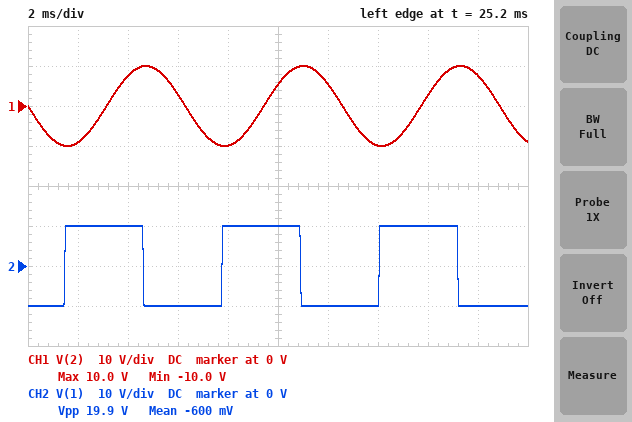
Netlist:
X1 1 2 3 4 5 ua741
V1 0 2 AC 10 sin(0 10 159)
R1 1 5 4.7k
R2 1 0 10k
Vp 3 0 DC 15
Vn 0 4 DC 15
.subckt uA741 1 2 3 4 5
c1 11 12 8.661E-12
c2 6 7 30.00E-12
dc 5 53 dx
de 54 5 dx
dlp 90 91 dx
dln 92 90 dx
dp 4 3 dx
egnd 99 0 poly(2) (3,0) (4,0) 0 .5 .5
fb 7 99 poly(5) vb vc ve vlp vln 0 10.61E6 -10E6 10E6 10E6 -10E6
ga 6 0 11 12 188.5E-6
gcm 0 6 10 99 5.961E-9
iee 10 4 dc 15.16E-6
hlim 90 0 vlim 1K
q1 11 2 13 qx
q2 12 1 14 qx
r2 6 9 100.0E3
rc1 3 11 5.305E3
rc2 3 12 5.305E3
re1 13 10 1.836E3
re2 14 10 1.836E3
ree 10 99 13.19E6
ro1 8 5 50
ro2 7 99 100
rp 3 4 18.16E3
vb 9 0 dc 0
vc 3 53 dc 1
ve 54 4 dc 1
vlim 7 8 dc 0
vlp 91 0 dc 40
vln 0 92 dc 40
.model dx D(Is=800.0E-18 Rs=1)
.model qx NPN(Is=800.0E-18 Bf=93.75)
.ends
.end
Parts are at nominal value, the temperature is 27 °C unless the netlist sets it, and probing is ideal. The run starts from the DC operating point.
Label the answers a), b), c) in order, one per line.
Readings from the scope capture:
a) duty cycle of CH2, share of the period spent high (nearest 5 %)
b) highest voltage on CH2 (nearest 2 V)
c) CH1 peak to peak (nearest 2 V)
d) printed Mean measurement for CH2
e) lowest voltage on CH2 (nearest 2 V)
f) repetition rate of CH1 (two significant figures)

a) 50 %
b) 10 V
c) 20 V
d) -600 mV
e) -10 V
f) 160 Hz
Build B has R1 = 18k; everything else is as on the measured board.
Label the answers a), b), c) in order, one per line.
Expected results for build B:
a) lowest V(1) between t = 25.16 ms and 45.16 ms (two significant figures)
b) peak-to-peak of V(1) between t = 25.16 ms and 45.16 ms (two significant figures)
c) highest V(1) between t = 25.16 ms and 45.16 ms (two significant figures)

a) -5.2 V
b) 10 V
c) 5.2 V
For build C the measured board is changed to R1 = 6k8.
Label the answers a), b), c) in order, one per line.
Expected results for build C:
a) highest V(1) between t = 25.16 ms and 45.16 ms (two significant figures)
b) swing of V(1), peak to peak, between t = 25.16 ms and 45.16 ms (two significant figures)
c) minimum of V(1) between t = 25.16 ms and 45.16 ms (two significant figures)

a) 8.7 V
b) 17 V
c) -8.7 V
